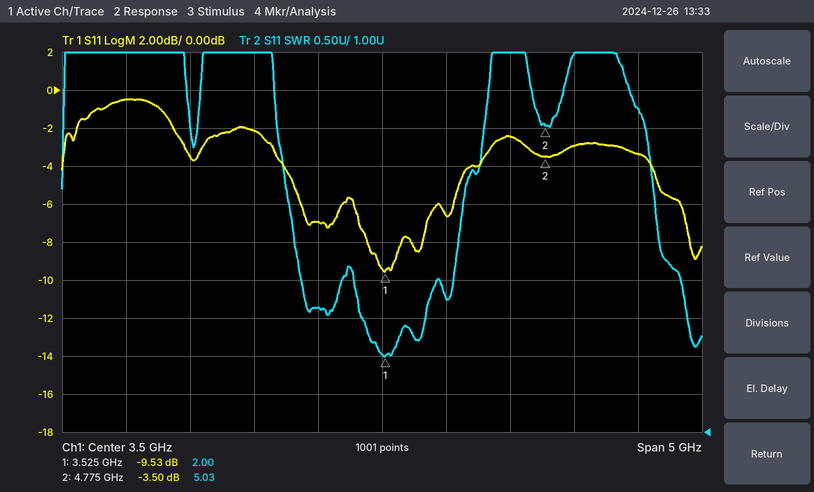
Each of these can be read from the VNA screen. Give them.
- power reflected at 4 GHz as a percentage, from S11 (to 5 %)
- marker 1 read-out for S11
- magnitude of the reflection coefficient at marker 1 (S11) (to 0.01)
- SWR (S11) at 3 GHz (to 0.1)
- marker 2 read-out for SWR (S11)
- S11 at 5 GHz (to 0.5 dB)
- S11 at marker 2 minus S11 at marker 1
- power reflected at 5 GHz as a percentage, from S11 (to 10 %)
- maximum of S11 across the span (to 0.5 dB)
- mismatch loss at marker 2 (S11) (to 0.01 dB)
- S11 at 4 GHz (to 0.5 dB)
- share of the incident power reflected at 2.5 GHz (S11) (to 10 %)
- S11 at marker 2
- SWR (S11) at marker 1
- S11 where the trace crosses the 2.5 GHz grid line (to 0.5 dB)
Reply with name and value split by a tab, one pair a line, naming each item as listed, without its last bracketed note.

power reflected at 4 GHz as a percentage, from S11	20 %
marker 1 read-out for S11	-9.53 dB
magnitude of the reflection coefficient at marker 1 (S11)	0.33
SWR (S11) at 3 GHz	2.6
marker 2 read-out for SWR	5.03
S11 at 5 GHz	-3.0 dB
S11 at marker 2 minus S11 at marker 1	6.03 dB
power reflected at 5 GHz as a percentage, from S11	50 %
maximum of S11 across the span	-0.5 dB
mismatch loss at marker 2 (S11)	2.57 dB
S11 at 4 GHz	-6.5 dB
share of the incident power reflected at 2.5 GHz (S11)	60 %
S11 at marker 2	-3.50 dB
SWR (S11) at marker 1	2.00
S11 where the trace crosses the 2.5 GHz grid line	-2.0 dB
